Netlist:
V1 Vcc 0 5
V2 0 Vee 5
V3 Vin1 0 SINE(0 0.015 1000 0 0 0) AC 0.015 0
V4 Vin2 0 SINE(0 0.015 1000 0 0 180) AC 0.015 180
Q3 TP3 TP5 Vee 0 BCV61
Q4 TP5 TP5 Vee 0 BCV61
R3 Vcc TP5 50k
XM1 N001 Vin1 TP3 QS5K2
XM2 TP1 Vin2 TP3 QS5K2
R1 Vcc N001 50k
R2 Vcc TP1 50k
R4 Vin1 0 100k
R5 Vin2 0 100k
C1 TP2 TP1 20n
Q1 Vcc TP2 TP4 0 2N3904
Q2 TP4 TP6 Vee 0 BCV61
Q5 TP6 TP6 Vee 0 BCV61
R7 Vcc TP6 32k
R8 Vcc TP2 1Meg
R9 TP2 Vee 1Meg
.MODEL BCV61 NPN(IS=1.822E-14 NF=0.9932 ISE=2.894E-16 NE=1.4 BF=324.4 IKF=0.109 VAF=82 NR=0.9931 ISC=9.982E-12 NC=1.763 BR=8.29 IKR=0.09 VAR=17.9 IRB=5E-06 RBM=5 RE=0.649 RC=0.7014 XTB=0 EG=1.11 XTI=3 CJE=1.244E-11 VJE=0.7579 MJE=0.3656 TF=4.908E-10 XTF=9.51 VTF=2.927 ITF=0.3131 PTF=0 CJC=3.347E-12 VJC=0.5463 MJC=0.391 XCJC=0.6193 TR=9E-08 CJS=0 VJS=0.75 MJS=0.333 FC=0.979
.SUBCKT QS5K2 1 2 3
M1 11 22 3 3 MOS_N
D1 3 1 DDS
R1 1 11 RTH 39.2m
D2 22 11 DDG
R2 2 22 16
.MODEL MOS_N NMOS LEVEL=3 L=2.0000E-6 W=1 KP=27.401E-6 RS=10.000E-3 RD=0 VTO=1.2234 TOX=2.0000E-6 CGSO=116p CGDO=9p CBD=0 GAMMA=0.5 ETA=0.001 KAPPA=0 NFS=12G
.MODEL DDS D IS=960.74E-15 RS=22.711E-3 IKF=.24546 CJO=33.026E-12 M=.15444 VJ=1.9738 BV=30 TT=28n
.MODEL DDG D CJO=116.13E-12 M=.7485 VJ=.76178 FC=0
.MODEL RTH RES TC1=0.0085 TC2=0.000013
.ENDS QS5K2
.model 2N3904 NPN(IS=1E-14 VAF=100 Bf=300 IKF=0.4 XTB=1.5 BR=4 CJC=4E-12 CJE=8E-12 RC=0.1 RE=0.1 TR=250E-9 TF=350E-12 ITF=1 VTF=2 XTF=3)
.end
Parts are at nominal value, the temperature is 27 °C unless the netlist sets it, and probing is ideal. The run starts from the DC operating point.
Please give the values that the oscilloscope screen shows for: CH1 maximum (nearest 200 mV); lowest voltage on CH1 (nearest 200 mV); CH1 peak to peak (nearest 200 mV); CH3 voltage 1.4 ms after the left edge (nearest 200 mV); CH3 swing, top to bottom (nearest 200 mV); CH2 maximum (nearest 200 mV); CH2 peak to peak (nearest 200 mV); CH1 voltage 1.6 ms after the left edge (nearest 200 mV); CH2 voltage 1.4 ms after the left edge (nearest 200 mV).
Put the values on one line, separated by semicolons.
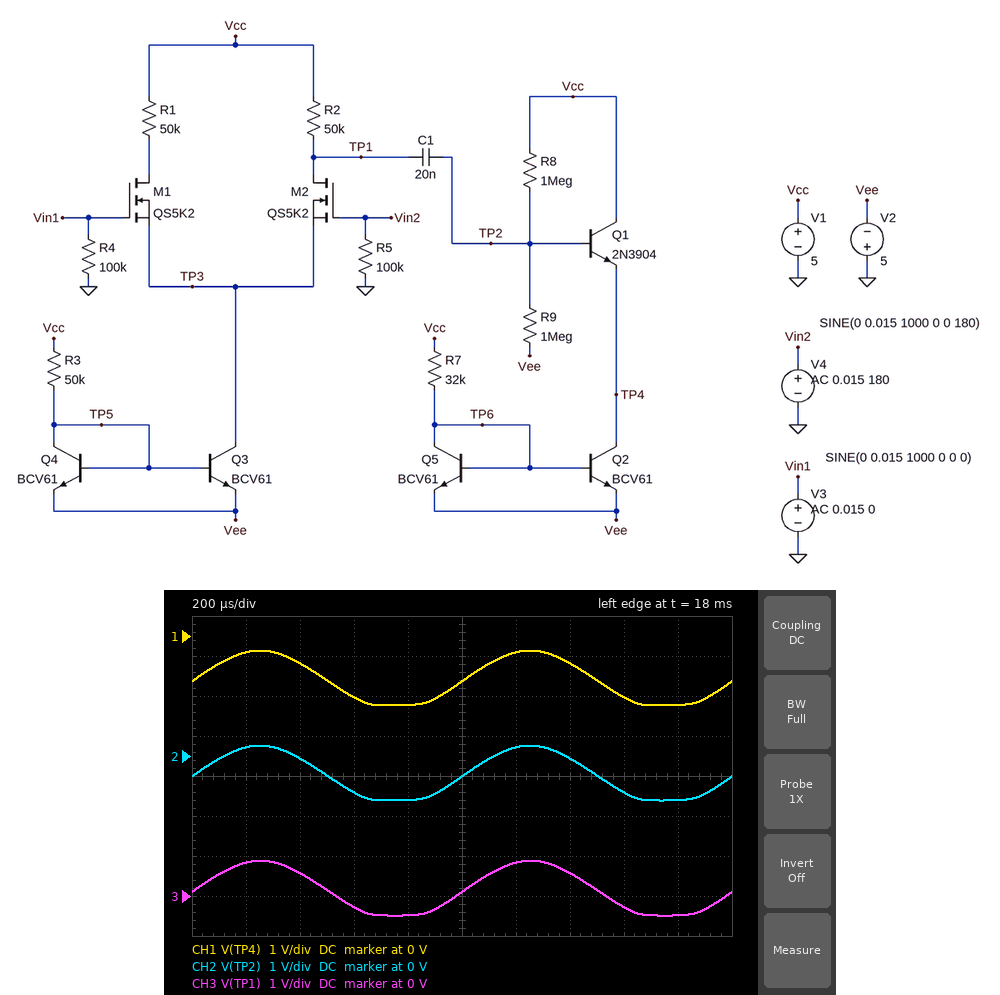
-400 mV; -1.8 V; 1.4 V; 600 mV; 1.4 V; 200 mV; 1.4 V; -1.6 V; 0 V
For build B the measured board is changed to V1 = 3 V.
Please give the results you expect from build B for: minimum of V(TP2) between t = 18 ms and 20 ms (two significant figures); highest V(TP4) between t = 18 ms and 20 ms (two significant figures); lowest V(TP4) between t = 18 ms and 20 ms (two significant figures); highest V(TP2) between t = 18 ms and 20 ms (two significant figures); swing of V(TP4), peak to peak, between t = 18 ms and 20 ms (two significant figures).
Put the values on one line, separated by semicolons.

-1.5 V; -1.6 V; -2.1 V; -1.0 V; 470 mV
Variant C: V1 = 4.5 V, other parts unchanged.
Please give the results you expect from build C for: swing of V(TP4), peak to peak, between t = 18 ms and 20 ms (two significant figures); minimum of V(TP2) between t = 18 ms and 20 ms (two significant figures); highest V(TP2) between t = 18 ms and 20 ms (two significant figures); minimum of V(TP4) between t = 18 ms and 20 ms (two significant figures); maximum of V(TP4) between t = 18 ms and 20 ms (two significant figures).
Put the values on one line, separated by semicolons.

1.2 V; -1.2 V; -11 mV; -1.8 V; -630 mV
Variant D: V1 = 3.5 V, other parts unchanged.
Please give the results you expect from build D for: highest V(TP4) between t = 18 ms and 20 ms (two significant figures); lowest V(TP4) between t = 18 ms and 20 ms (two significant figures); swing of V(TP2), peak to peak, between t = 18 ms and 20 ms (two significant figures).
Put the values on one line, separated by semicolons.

-1.3 V; -2.0 V; 710 mV
